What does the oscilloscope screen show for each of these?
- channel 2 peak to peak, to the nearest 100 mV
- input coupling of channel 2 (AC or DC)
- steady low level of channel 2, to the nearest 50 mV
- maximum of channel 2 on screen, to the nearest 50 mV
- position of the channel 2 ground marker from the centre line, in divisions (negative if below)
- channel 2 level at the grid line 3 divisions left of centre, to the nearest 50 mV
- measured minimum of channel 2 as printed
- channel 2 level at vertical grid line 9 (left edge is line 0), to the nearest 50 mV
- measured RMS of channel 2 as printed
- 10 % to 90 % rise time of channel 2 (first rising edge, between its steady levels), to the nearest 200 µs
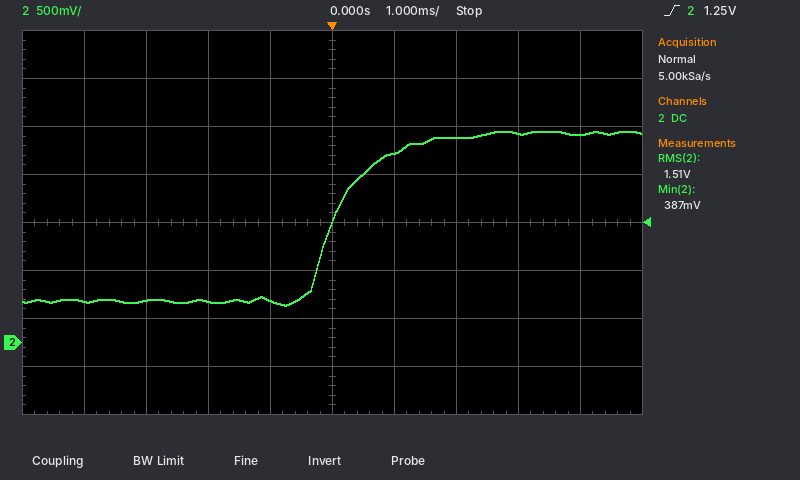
1.80 V
DC
450 mV
2.20 V
-2.5 div
450 mV
387 mV
2.15 V
1.51 V
1.4 ms
